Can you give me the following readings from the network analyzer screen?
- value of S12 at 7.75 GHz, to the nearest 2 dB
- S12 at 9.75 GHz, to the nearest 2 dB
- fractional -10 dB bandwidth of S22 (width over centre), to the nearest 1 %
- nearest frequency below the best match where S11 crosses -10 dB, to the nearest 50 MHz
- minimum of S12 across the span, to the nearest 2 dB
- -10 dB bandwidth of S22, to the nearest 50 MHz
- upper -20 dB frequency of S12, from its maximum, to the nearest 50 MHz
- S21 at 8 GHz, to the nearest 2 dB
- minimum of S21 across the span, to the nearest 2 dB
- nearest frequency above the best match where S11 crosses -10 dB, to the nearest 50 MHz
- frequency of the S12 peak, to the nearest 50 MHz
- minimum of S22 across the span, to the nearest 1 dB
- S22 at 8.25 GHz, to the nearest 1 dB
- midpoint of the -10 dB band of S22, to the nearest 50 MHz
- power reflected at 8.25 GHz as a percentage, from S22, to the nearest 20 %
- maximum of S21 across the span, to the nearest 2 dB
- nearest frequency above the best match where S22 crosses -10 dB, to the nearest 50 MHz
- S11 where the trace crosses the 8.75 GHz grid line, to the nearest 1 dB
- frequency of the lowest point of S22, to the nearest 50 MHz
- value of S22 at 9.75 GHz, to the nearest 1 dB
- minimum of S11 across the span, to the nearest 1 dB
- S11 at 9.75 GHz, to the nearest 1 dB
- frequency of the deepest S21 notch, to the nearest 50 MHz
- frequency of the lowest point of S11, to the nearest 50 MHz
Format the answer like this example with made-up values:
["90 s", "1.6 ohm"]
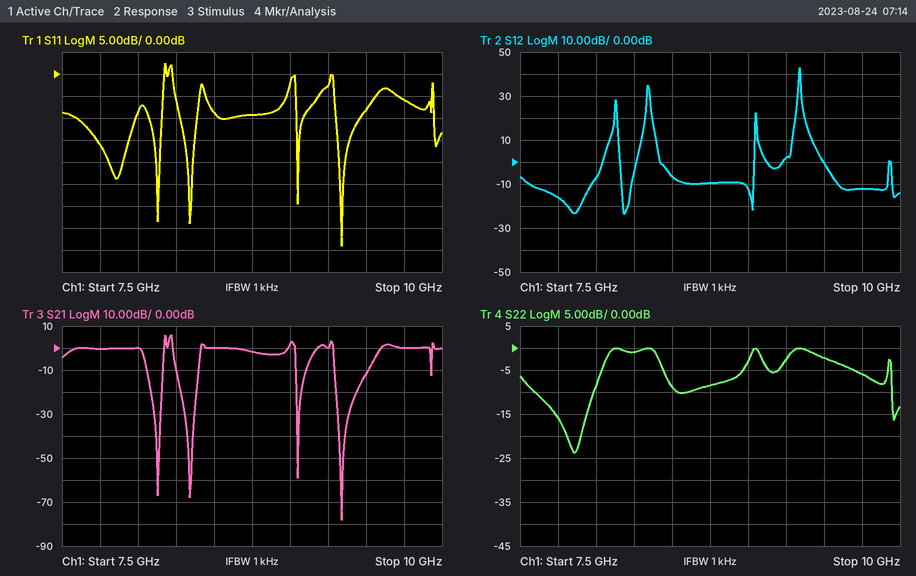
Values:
["-16 dB", "-12 dB", "5 %", "9.30 GHz", "-24 dB", "400 MHz", "9.35 GHz", "0 dB", "-78 dB", "9.45 GHz", "9.35 GHz", "-24 dB", "-1 dB", "7.80 GHz", "80 %", "6 dB", "8.00 GHz", "-9 dB", "7.85 GHz", "-6 dB", "-39 dB", "-6 dB", "9.35 GHz", "9.35 GHz"]
